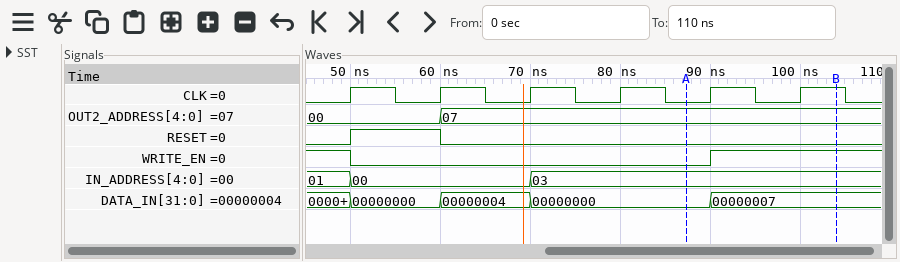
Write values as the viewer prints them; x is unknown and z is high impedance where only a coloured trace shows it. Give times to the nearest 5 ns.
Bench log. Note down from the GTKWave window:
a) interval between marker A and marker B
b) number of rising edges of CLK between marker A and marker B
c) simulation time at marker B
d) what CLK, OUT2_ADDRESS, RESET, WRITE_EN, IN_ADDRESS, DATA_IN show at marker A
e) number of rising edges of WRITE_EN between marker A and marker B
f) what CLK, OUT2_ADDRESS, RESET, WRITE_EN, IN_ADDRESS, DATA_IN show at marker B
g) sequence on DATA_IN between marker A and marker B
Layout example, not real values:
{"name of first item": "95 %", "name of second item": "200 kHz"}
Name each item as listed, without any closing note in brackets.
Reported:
{"interval between marker A and marker B": "15 ns", "number of rising edges of CLK between marker A and marker B": "2", "simulation time at marker B": "105 ns", "what CLK, OUT2_ADDRESS, RESET, WRITE_EN, IN_ADDRESS, DATA_IN show at marker A": "CLK=0, OUT2_ADDRESS=07, RESET=0, WRITE_EN=0, IN_ADDRESS=03, DATA_IN=00000000", "number of rising edges of WRITE_EN between marker A and marker B": "1", "what CLK, OUT2_ADDRESS, RESET, WRITE_EN, IN_ADDRESS, DATA_IN show at marker B": "CLK=1, OUT2_ADDRESS=07, RESET=0, WRITE_EN=1, IN_ADDRESS=03, DATA_IN=00000007", "sequence on DATA_IN between marker A and marker B": "00000000, 00000007"}
